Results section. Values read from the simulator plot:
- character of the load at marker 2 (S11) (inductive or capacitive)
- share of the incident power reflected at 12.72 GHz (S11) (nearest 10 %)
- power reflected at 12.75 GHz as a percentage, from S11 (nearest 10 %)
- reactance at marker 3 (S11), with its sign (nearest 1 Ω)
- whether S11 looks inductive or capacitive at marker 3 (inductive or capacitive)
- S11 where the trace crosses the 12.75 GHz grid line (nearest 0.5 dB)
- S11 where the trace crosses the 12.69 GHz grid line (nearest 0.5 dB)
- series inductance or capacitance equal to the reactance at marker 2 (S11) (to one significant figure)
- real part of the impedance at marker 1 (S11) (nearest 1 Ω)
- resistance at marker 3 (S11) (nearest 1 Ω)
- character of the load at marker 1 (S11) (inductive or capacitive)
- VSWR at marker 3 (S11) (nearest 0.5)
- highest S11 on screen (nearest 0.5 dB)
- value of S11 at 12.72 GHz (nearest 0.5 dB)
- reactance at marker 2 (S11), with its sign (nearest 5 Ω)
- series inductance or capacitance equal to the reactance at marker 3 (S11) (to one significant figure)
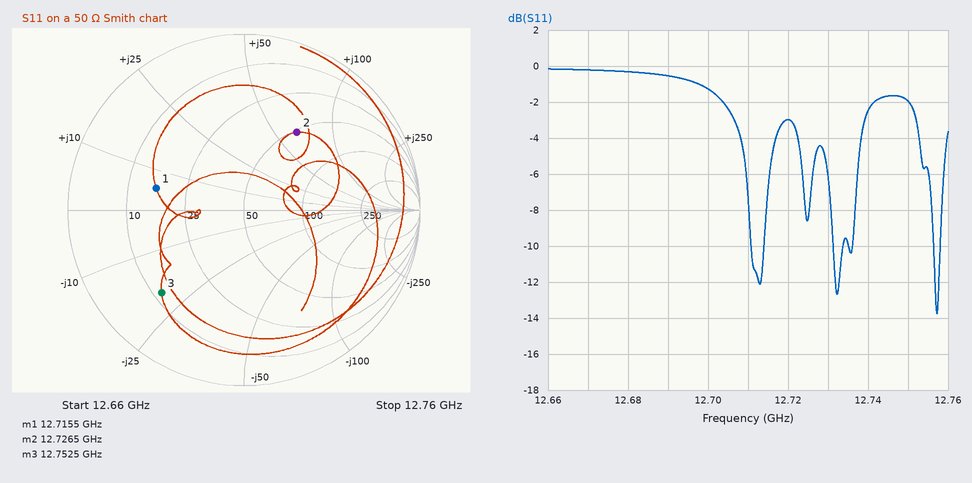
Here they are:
inductive
50 %
60 %
-20 Ω
capacitive
-2.0 dB
-0.5 dB
800 pH
16 Ω
12 Ω
inductive
5.0
0.0 dB
-3.0 dB
+65 Ω
600 fF
